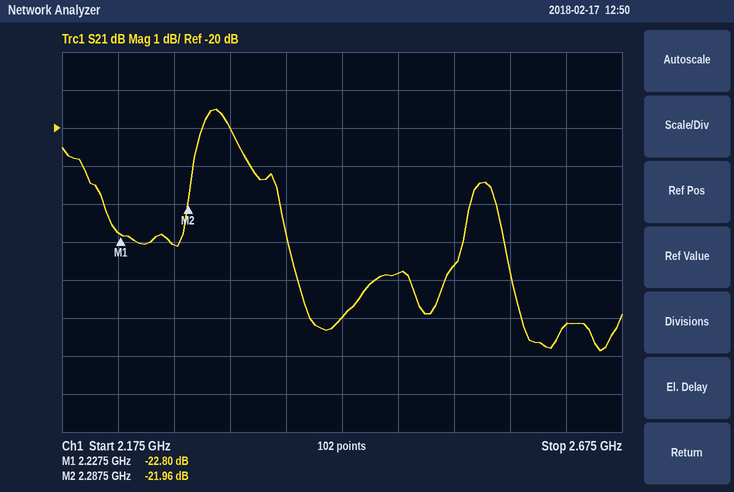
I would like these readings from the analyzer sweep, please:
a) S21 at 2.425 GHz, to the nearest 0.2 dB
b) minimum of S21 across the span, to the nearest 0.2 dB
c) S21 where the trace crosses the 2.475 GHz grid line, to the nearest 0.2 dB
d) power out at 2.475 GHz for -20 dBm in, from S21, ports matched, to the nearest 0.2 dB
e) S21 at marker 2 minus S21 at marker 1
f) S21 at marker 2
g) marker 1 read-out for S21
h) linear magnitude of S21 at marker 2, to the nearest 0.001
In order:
-25.0 dB
-25.8 dB
-23.8 dB
-43.8 dBm
0.84 dB
-21.96 dB
-22.80 dB
0.080
